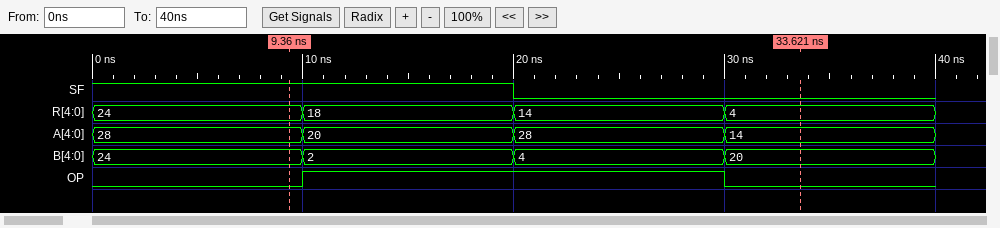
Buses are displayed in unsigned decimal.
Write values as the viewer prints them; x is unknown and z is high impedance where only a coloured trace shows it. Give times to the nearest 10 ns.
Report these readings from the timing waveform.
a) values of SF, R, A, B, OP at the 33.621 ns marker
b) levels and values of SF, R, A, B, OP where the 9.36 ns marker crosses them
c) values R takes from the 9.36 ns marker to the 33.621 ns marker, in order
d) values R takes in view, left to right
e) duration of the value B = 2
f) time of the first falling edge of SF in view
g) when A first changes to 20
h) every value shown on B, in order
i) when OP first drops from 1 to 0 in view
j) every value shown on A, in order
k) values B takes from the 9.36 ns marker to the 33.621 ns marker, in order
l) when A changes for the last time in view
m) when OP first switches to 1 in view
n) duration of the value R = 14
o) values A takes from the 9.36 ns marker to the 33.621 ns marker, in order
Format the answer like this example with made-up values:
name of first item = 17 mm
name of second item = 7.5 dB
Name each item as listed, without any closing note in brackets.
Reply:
values of SF, R, A, B, OP at the 33.621 ns marker = SF=0, R=4, A=14, B=20, OP=0
levels and values of SF, R, A, B, OP where the 9.36 ns marker crosses them = SF=1, R=24, A=28, B=24, OP=0
values R takes from the 9.36 ns marker to the 33.621 ns marker, in order = 24, 18, 14, 4
values R takes in view, left to right = 24, 18, 14, 4
duration of the value B = 2 = 10 ns
time of the first falling edge of SF in view = 20 ns
when A first changes to 20 = 10 ns
every value shown on B, in order = 24, 2, 4, 20
when OP first drops from 1 to 0 in view = 30 ns
every value shown on A, in order = 28, 20, 28, 14
values B takes from the 9.36 ns marker to the 33.621 ns marker, in order = 24, 2, 4, 20
when A changes for the last time in view = 30 ns
when OP first switches to 1 in view = 10 ns
duration of the value R = 14 = 10 ns
values A takes from the 9.36 ns marker to the 33.621 ns marker, in order = 28, 20, 28, 14
